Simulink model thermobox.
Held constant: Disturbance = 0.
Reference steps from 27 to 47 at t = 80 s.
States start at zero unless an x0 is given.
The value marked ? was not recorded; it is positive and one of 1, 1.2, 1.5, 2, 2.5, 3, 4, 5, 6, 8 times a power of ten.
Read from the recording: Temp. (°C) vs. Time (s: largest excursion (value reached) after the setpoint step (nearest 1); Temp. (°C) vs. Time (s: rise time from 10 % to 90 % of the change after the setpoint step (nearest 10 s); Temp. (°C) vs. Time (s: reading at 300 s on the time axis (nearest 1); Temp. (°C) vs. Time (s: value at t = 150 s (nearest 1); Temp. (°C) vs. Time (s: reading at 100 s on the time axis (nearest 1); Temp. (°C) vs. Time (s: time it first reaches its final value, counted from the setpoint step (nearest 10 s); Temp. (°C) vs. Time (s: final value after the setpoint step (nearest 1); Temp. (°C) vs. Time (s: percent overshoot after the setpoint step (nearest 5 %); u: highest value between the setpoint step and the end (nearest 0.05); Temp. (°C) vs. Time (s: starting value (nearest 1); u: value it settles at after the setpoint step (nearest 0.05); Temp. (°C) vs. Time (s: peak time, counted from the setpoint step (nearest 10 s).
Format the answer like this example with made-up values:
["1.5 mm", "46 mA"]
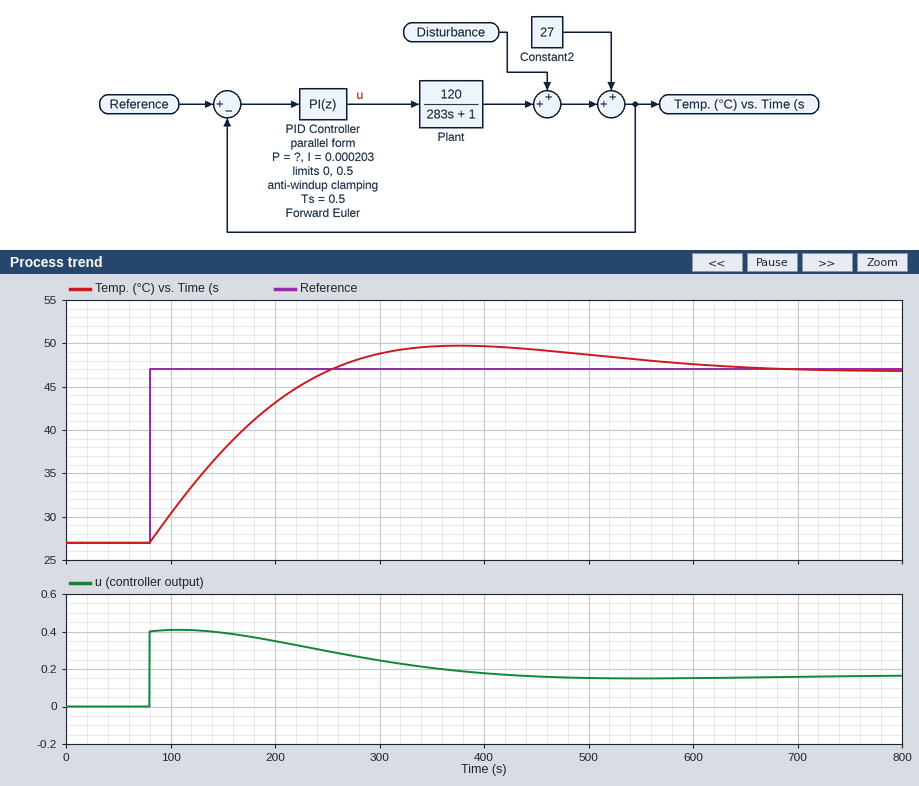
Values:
["50", "130 s", "49", "38", "30", "170 s", "47", "15 %", "0.40", "27", "0.15", "300 s"]
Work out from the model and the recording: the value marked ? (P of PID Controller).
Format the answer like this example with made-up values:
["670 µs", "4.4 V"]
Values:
["0.02"]
